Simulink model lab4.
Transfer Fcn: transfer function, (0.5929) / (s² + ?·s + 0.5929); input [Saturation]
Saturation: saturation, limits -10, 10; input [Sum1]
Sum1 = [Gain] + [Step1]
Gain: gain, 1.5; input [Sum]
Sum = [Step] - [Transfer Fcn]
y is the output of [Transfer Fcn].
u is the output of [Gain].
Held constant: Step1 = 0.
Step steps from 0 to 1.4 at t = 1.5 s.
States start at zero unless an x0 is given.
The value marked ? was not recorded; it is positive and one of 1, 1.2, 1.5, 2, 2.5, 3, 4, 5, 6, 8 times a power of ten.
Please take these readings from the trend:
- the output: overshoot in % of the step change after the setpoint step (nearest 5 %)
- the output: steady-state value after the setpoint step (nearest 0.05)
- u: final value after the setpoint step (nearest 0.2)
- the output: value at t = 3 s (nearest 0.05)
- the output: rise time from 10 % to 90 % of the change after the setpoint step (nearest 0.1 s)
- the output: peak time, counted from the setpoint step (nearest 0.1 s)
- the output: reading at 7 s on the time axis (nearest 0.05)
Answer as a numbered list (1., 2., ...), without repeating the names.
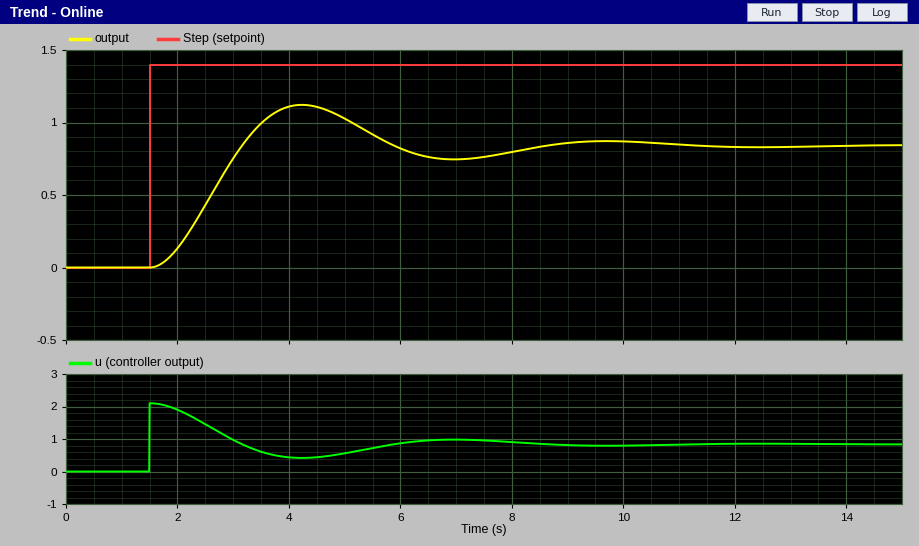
1. 35 %
2. 0.85
3. 0.8
4. 0.75
5. 1.1 s
6. 2.7 s
7. 0.75
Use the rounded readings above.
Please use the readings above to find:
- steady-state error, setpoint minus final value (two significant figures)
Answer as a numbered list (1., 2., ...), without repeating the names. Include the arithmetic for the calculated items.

1. 1.4 - 0.85 = 0.55
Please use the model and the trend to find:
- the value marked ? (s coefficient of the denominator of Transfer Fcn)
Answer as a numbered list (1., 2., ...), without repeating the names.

1. 0.8
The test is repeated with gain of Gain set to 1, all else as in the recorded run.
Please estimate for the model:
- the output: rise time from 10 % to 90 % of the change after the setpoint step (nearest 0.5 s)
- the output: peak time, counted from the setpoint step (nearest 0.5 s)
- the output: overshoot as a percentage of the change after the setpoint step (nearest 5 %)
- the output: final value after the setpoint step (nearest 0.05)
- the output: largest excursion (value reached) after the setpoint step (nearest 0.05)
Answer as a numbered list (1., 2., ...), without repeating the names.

1. 1.5 s
2. 3.0 s
3. 30 %
4. 0.70
5. 0.90
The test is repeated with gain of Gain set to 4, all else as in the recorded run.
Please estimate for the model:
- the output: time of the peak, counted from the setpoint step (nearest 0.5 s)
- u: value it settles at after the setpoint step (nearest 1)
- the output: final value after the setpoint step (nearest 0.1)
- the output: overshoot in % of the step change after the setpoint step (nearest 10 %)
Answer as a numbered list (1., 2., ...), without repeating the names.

1. 2.0 s
2. 1
3. 1.1
4. 50 %
